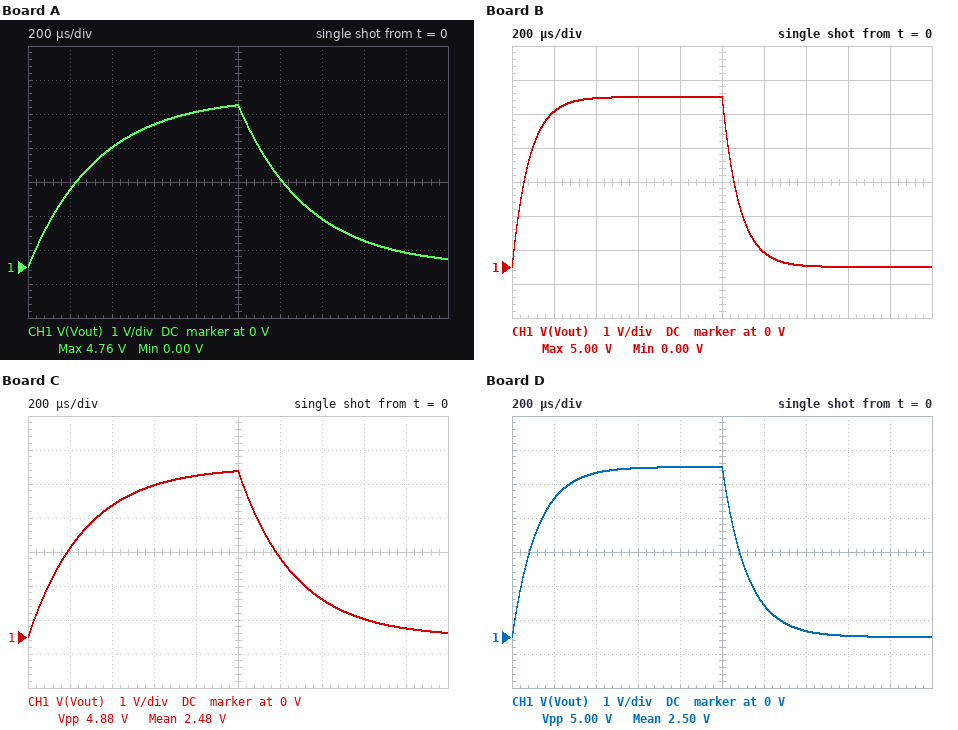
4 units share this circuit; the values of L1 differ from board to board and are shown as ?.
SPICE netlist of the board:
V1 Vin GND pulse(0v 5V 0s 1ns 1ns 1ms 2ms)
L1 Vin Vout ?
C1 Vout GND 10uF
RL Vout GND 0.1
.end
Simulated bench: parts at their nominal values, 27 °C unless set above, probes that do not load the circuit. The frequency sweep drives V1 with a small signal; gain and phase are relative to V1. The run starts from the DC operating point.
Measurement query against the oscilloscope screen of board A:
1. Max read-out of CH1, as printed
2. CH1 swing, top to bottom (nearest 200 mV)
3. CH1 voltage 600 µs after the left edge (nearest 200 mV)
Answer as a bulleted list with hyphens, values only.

- 4.76 V
- 4.8 V
- 4.2 V
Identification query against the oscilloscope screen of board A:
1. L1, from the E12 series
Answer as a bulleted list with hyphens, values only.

- 33 µH
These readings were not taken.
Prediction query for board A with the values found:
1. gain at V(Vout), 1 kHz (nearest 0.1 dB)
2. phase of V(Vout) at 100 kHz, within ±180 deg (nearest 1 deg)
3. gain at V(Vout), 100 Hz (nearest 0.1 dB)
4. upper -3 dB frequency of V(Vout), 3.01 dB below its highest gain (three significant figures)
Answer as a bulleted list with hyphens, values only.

- -7.2 dB
- -122 deg
- -0.2 dB
- 484 Hz
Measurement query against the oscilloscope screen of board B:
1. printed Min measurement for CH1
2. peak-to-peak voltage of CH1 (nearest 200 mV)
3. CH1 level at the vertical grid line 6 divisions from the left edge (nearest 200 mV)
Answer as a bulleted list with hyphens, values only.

- 0.00 V
- 5.0 V
- 400 mV
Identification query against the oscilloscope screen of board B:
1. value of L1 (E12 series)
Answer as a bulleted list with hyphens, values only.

- 8.2 µH
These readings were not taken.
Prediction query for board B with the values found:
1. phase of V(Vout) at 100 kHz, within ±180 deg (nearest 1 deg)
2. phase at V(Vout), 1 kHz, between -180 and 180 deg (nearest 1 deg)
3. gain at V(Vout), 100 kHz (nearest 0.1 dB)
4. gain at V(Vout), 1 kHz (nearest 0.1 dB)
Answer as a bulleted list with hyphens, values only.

- -121 deg
- -27 deg
- -35.6 dB
- -1.0 dB
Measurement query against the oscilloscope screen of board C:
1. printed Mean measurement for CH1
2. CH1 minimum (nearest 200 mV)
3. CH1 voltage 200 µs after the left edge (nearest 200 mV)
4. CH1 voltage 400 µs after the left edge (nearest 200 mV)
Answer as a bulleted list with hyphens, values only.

- 2.48 V
- 0 V
- 2.6 V
- 3.8 V
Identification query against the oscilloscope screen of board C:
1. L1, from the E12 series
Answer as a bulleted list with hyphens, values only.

- 27 µH
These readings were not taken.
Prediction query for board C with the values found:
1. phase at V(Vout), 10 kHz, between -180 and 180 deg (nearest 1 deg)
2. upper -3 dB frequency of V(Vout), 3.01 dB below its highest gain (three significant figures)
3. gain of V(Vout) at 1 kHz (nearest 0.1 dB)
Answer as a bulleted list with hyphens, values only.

- -90 deg
- 592 Hz
- -5.9 dB
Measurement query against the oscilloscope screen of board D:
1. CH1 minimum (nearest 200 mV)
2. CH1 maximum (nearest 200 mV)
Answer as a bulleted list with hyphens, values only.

- 0 V
- 5.0 V
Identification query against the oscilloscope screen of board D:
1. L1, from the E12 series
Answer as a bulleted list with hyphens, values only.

- 12 µH
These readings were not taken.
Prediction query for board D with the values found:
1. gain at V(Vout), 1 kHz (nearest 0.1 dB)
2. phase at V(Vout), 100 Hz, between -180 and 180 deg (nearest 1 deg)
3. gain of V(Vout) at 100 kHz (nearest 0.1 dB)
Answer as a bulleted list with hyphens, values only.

- -1.9 dB
- -4 deg
- -38.9 dB
